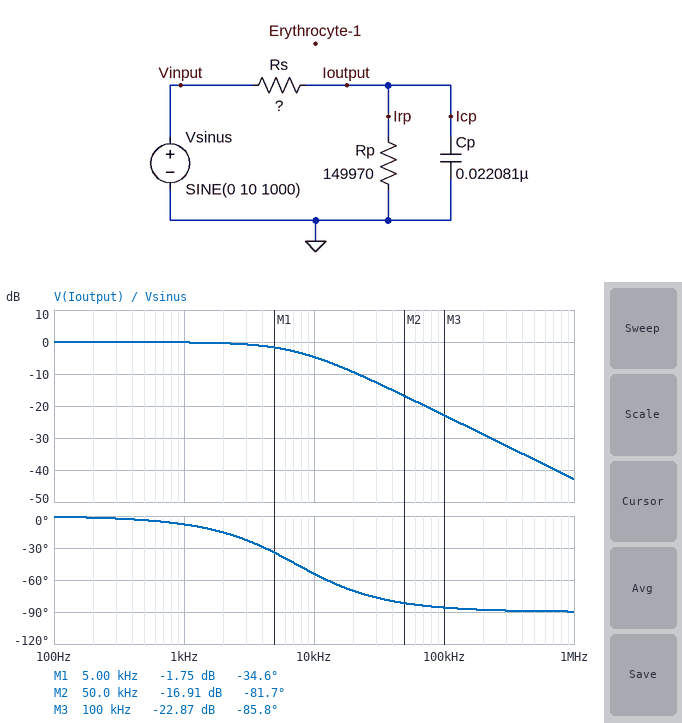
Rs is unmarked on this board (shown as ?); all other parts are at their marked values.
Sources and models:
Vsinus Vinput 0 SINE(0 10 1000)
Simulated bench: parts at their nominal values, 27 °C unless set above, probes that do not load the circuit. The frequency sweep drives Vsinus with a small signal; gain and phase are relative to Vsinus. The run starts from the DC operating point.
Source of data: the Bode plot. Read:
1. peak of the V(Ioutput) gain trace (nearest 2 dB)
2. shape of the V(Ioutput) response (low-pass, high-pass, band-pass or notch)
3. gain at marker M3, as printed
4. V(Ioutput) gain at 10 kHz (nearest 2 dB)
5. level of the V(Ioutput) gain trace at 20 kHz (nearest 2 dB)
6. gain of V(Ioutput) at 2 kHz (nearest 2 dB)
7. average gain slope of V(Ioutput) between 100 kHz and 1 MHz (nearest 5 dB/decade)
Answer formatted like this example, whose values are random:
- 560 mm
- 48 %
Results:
- 0 dB
- low-pass
- -22.87 dB
- -4 dB
- -10 dB
- 0 dB
- -20 dB/decade
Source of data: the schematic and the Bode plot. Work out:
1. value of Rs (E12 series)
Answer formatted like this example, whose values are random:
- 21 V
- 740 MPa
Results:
- 1 kΩ
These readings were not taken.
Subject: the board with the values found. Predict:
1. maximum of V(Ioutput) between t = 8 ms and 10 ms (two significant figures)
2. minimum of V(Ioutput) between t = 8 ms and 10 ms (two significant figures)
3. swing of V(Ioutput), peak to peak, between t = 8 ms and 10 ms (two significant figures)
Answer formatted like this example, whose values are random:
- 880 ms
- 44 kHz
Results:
- 9.8 V
- -9.8 V
- 20 V
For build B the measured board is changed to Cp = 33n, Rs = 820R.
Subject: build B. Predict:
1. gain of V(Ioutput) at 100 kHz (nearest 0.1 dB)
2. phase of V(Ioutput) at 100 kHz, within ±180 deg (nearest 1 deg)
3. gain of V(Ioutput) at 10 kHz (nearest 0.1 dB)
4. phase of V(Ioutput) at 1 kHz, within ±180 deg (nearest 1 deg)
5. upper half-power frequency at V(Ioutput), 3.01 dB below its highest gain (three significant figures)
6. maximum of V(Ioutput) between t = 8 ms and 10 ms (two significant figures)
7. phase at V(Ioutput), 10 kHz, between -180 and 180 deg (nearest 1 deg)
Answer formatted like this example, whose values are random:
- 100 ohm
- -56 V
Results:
- -24.6 dB
- -87 deg
- -5.9 dB
- -10 deg
- 5.91 kHz
- 9.8 V
- -59 deg
